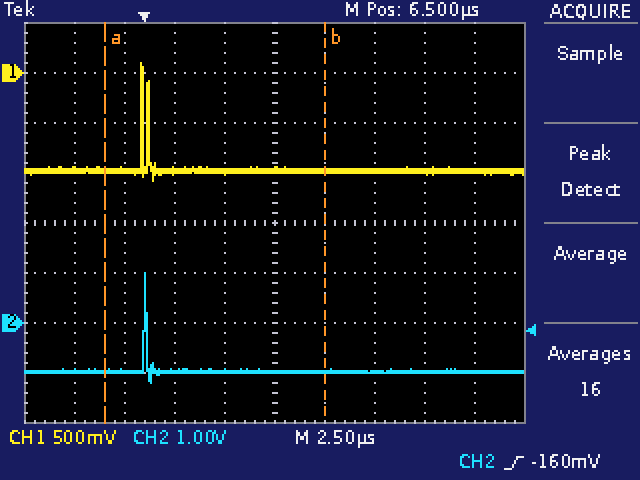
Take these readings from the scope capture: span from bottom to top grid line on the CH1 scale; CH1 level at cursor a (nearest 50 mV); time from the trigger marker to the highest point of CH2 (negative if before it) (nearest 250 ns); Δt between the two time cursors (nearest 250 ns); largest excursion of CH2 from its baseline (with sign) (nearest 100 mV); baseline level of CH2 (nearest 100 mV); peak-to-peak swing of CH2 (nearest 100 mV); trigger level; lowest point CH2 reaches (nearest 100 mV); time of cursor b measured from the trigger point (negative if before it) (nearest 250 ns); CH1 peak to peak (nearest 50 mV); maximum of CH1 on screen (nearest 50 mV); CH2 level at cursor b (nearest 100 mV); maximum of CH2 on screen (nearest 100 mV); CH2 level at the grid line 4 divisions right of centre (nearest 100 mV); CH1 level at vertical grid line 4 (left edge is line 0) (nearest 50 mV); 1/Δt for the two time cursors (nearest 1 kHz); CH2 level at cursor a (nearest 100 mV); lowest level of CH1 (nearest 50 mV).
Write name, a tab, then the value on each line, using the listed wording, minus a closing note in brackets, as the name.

span from bottom to top grid line on the CH1 scale	4 V
CH1 level at cursor a	-950 mV
time from the trigger marker to the highest point of CH2 (negative if before it)	0.00 µs
Δt between the two time cursors	11.00 µs
largest excursion of CH2 from its baseline (with sign)	+2.0 V
baseline level of CH2	-1.0 V
peak-to-peak swing of CH2	2.2 V
trigger level	-160 mV
lowest point CH2 reaches	-1.2 V
time of cursor b measured from the trigger point (negative if before it)	+9.00 µs
CH1 peak to peak	1.20 V
maximum of CH1 on screen	100 mV
CH2 level at cursor b	-1.0 V
maximum of CH2 on screen	1.0 V
CH2 level at the grid line 4 divisions right of centre	-1.0 V
CH1 level at vertical grid line 4 (left edge is line 0)	-1.00 V
1/Δt for the two time cursors	91 kHz
CH2 level at cursor a	-1.0 V
lowest level of CH1	-1.10 V
